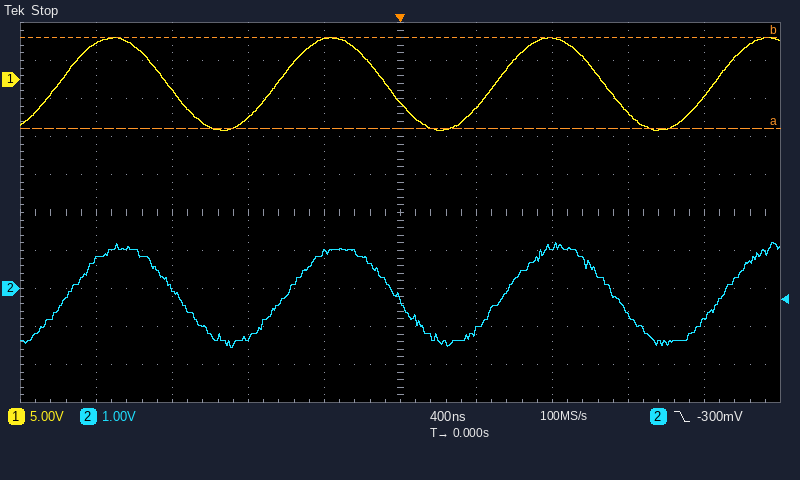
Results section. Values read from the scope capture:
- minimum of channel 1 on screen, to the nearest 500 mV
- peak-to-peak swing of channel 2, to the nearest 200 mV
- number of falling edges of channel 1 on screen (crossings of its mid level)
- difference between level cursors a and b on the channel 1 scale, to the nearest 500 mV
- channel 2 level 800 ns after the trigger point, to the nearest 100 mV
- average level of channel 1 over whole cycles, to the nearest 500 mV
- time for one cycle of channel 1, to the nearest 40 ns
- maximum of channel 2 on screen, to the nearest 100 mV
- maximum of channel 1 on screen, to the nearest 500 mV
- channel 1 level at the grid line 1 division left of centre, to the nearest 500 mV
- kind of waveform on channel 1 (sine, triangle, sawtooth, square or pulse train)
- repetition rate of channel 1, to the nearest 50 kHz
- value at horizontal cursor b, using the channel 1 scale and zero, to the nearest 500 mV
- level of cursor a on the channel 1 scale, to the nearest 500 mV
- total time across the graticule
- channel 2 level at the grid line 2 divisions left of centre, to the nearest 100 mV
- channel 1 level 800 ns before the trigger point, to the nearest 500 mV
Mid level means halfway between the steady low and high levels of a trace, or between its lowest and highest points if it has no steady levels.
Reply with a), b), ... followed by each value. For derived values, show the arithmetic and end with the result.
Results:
a) -6.5 V
b) 2.8 V
c) 3
d) 12.0 V
e) 1.1 V
f) (5.5 V + (-6.5 V)) / 2 ≈ -500 mV
g) 1.16 µs
h) 1.2 V
i) 5.5 V
j) 5.5 V
k) sine
l) 1 / 1.16 µs ≈ 862 kHz, so 850 kHz to the nearest 50 kHz
m) 5.5 V
n) -6.5 V
o) 4 µs
p) -1.3 V
q) -5.0 V
